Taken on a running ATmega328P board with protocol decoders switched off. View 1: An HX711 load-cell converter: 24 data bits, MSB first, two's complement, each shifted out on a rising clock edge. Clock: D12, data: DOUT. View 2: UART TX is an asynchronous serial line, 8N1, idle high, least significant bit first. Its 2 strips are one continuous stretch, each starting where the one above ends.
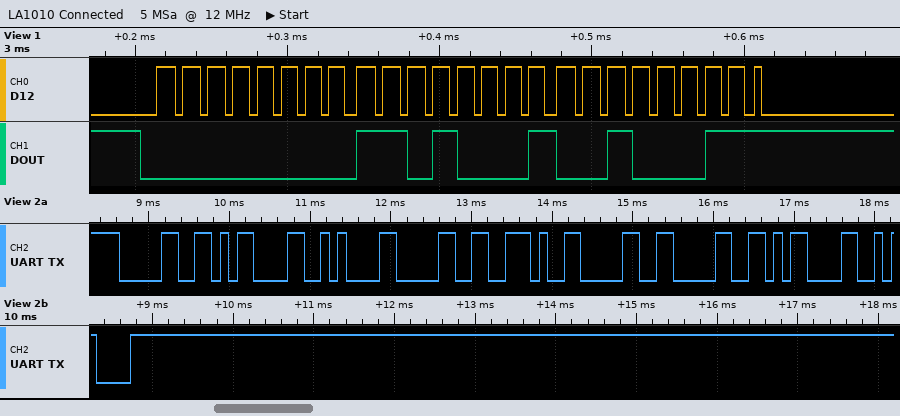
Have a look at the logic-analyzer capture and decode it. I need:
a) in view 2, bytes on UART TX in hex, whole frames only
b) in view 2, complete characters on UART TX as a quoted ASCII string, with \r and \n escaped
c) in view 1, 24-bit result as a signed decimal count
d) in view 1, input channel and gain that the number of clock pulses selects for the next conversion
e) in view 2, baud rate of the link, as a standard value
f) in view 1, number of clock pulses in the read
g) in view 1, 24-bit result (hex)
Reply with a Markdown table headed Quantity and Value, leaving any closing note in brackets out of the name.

| Quantity | Value |
|---|---|
| in view 2, bytes on UART TX in hex, whole frames only | 30 0D 0A 30 2E 30 30 0D 0A |
| in view 2, complete characters on UART TX as a quoted ASCII string, with \r and \n escaped | "0\r\n0.00\r\n" |
| in view 1, 24-bit result as a signed decimal count | 53539 |
| in view 1, input channel and gain that the number of clock pulses selects for the next conversion | channel A, gain 128 |
| in view 2, baud rate of the link, as a standard value | 9600 baud |
| in view 1, number of clock pulses in the read | 25 |
| in view 1, 24-bit result | 0x00D123 |
